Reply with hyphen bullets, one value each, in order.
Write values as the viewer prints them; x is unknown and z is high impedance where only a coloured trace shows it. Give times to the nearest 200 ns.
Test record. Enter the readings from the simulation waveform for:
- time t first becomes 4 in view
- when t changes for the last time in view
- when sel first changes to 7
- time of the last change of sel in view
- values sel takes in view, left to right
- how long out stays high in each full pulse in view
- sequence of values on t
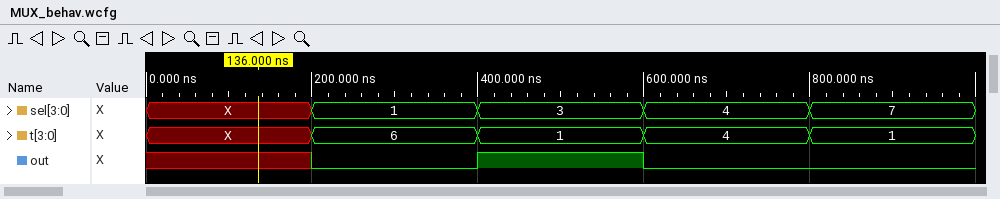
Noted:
- 600 ns
- 800 ns
- 800 ns
- 800 ns
- X, 1, 3, 4, 7
- 200 ns
- X, 6, 1, 4, 1
